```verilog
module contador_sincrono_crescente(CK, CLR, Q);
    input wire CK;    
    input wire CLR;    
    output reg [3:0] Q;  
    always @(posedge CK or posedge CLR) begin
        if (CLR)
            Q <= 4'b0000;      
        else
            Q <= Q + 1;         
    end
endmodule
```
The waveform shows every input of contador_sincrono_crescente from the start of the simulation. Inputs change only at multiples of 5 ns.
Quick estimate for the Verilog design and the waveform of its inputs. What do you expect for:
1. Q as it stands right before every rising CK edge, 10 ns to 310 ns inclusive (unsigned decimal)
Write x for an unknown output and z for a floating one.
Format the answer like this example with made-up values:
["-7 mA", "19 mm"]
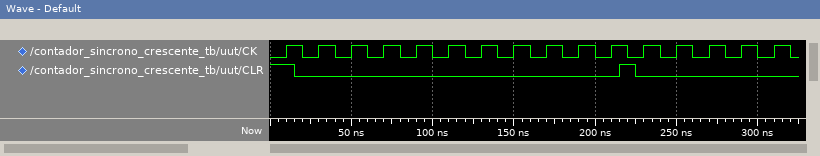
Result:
["0, 0, 1, 2, 3, 4, 5, 6, 7, 8, 9, 0, 1, 2, 3, 4"]
